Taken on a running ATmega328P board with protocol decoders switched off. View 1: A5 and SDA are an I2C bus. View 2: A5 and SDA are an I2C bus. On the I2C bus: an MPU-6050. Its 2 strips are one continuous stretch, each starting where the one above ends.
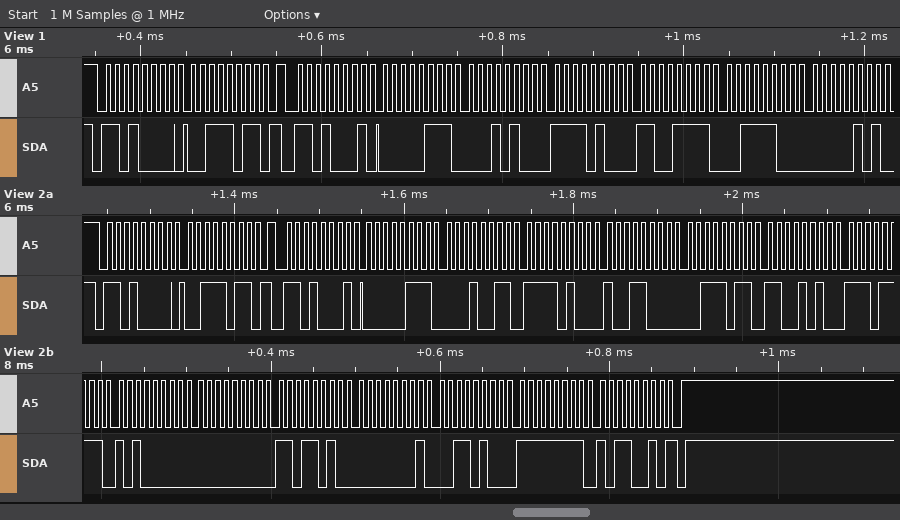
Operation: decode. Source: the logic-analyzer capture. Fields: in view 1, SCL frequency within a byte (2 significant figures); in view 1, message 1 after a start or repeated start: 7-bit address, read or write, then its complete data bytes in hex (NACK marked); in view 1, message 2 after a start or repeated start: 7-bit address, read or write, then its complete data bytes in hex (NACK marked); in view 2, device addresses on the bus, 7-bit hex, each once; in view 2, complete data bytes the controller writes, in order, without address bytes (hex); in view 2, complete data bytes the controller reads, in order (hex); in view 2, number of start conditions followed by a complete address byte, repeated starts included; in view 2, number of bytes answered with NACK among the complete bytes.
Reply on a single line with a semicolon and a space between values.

100 kHz; 0x68 write: 3B; 0x68 read: 07 14 F4 CF 3C 05; 0x68; 3B; 07 13 F4 98 3B CA EF A0 00 DA 01 34 FF B2; 2; 1
